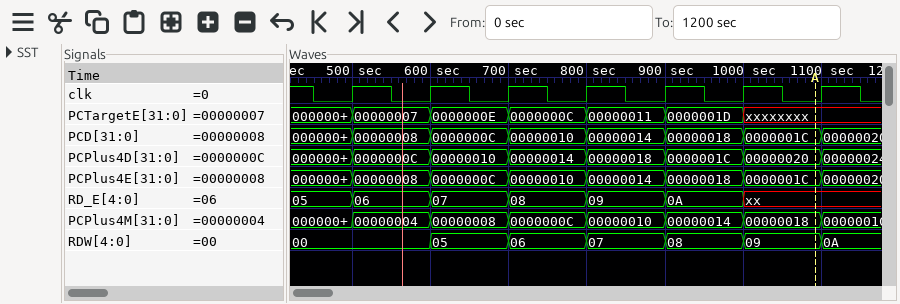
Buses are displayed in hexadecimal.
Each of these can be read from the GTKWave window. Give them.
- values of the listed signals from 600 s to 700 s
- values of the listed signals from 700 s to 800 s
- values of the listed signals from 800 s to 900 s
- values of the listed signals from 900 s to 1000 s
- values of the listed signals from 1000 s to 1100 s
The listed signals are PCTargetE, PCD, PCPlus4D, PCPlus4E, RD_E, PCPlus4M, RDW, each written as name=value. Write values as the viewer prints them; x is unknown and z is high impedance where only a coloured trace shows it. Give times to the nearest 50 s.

PCTargetE=0000000E, PCD=0000000C, PCPlus4D=00000010, PCPlus4E=0000000C, RD_E=07, PCPlus4M=00000008, RDW=05
PCTargetE=0000000C, PCD=00000010, PCPlus4D=00000014, PCPlus4E=00000010, RD_E=08, PCPlus4M=0000000C, RDW=06
PCTargetE=00000011, PCD=00000014, PCPlus4D=00000018, PCPlus4E=00000014, RD_E=09, PCPlus4M=00000010, RDW=07
PCTargetE=0000001D, PCD=00000018, PCPlus4D=0000001C, PCPlus4E=00000018, RD_E=0A, PCPlus4M=00000014, RDW=08
PCTargetE=xxxxxxxx, PCD=0000001C, PCPlus4D=00000020, PCPlus4E=0000001C, RD_E=xx, PCPlus4M=00000018, RDW=09
